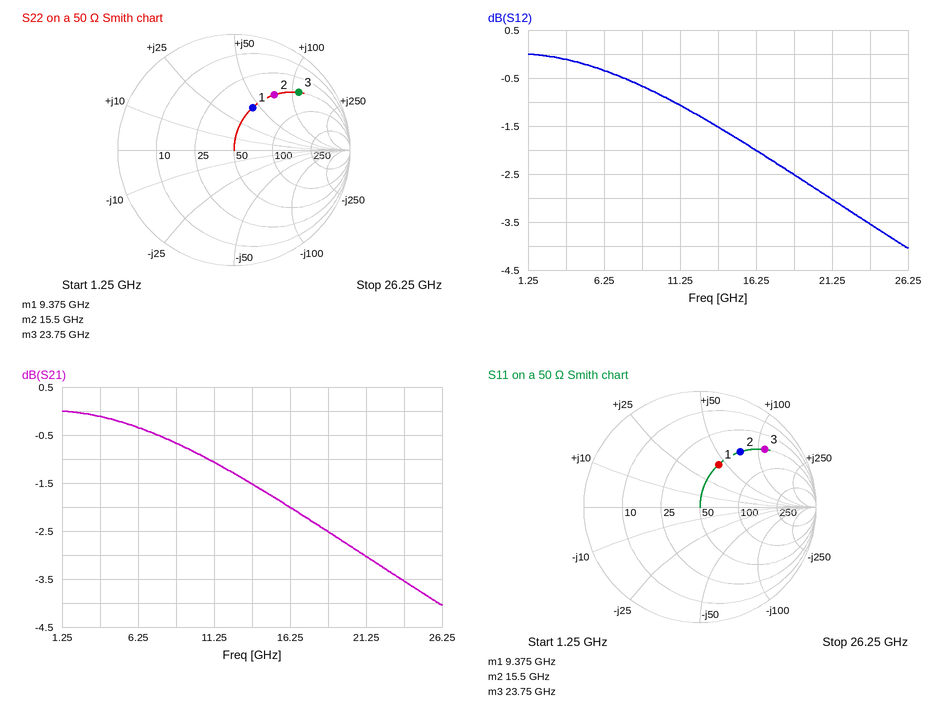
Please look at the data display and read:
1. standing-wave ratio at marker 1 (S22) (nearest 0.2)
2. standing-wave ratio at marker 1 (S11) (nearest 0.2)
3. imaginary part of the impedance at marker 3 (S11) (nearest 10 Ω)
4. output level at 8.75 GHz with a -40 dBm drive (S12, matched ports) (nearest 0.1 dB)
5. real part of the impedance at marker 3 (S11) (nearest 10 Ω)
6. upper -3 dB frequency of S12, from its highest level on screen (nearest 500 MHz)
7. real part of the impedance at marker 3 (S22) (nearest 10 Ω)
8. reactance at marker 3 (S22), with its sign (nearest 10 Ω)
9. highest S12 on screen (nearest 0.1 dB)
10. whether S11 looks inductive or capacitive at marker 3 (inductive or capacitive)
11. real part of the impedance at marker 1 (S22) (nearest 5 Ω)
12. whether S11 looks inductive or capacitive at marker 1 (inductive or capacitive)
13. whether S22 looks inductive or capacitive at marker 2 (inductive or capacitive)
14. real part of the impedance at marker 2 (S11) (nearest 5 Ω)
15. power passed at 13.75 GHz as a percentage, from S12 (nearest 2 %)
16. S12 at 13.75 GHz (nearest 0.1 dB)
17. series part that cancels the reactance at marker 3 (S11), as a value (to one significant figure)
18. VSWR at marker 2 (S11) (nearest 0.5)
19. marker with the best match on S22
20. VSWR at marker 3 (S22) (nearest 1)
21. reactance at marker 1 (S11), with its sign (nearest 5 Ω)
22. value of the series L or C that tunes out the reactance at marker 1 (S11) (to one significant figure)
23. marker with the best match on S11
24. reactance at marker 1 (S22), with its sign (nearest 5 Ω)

2.4
2.4
+110 Ω
-40.7 dBm
50 Ω
21.0 GHz
50 Ω
+110 Ω
0.0 dB
inductive
50 Ω
inductive
inductive
50 Ω
70 %
-1.5 dB
60 fF
4.0
marker 1
7
+45 Ω
400 fF
marker 1
+45 Ω
